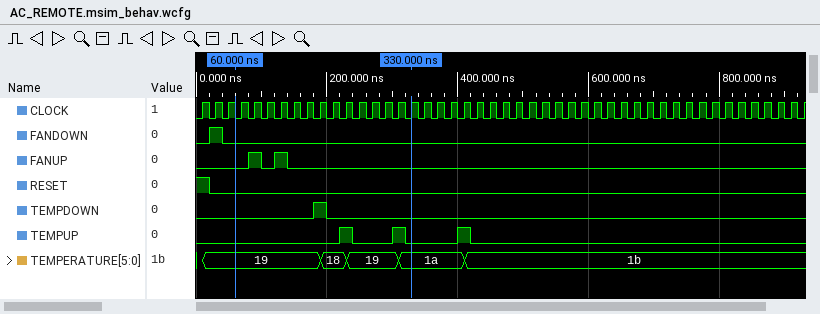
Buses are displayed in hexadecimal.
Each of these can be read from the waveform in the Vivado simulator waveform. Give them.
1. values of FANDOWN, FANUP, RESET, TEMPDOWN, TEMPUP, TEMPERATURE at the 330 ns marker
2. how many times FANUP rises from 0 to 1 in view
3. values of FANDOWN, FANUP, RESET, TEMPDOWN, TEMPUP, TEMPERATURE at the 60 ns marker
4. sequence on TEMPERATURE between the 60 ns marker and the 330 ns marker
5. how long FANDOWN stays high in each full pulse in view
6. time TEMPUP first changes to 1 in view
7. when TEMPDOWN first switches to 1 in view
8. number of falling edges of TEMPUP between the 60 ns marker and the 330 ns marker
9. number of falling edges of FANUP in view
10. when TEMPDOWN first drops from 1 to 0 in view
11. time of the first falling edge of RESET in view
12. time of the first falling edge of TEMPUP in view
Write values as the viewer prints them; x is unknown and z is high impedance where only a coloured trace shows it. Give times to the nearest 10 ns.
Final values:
FANDOWN=0, FANUP=0, RESET=0, TEMPDOWN=0, TEMPUP=0, TEMPERATURE=1a
2
FANDOWN=0, FANUP=0, RESET=0, TEMPDOWN=0, TEMPUP=0, TEMPERATURE=19
19, 18, 19, 1a
20 ns
220 ns
180 ns
2
2
200 ns
20 ns
240 ns
